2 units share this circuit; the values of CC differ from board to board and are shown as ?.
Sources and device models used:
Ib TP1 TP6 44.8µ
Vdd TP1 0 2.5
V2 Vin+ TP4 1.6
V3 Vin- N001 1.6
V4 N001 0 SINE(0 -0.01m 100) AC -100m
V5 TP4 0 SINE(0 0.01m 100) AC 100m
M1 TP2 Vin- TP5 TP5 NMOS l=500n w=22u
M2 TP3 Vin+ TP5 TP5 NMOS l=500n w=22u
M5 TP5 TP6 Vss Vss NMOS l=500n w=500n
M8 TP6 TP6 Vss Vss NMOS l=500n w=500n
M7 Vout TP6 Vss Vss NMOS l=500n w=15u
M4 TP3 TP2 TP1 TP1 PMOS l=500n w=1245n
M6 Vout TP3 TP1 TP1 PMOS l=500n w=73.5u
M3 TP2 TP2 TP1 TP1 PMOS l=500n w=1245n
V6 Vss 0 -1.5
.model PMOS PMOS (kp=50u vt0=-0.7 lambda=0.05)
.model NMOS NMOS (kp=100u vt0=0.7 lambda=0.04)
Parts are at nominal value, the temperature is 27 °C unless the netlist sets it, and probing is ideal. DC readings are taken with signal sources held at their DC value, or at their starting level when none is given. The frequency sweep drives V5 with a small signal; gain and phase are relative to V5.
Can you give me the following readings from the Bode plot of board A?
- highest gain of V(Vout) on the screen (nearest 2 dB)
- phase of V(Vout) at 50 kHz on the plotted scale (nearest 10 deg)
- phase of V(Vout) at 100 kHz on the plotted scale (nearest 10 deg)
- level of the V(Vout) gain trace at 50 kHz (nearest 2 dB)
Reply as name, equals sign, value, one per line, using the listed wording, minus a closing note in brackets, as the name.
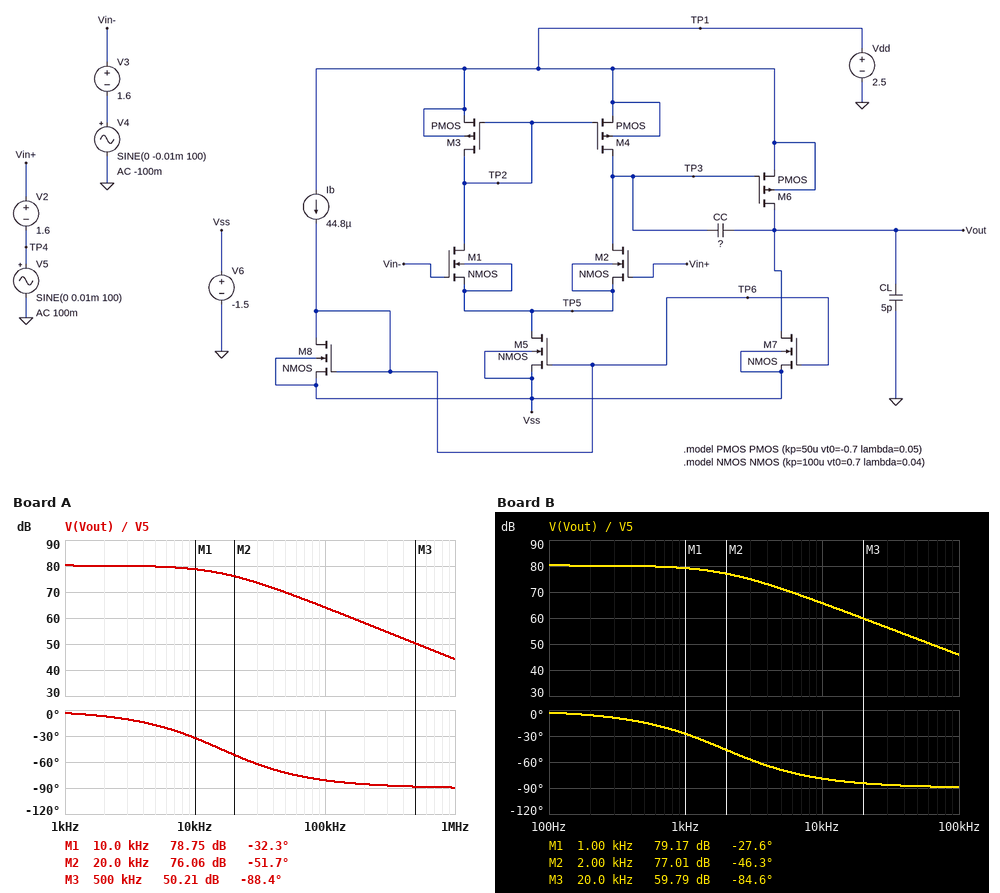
highest gain of V(Vout) on the screen = 80 dB
phase of V(Vout) at 50 kHz on the plotted scale = -70 deg
phase of V(Vout) at 100 kHz on the plotted scale = -80 deg
level of the V(Vout) gain trace at 50 kHz = 70 dB
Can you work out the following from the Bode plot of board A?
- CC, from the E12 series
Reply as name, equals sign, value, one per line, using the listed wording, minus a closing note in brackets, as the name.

CC, from the E12 series = 470 fF
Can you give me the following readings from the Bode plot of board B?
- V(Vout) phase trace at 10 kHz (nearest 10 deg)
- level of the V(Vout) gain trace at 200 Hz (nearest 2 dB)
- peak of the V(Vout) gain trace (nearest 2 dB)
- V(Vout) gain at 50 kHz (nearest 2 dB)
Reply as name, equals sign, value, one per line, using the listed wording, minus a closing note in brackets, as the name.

V(Vout) phase trace at 10 kHz = -80 deg
level of the V(Vout) gain trace at 200 Hz = 80 dB
peak of the V(Vout) gain trace = 80 dB
V(Vout) gain at 50 kHz = 52 dB
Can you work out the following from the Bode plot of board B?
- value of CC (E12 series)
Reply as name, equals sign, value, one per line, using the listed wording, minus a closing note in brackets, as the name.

value of CC = 3.9 pF
